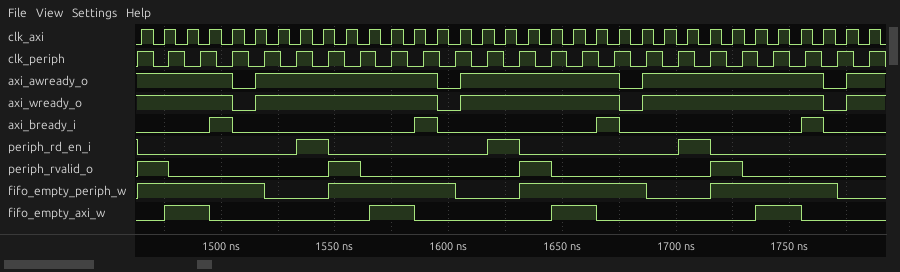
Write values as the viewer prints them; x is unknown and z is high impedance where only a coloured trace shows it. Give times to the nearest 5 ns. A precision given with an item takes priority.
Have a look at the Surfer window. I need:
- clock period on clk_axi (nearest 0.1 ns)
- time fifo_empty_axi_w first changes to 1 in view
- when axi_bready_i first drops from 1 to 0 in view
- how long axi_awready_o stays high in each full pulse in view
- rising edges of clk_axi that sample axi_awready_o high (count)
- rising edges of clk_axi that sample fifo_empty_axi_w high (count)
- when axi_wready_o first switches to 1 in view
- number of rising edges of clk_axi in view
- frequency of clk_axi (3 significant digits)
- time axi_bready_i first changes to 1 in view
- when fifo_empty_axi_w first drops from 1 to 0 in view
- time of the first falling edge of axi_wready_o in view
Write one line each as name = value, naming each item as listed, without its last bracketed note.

clock period on clk_axi = 10 ns
time fifo_empty_axi_w first changes to 1 in view = 1475 ns
when axi_bready_i first drops from 1 to 0 in view = 1505 ns
how long axi_awready_o stays high in each full pulse in view = 80 ns, 70 ns, 80 ns
rising edges of clk_axi that sample axi_awready_o high = 29
rising edges of clk_axi that sample fifo_empty_axi_w high = 8
when axi_wready_o first switches to 1 in view = 1515 ns
number of rising edges of clk_axi in view = 33
frequency of clk_axi = 100 MHz
time axi_bready_i first changes to 1 in view = 1495 ns
when fifo_empty_axi_w first drops from 1 to 0 in view = 1495 ns
time of the first falling edge of axi_wready_o in view = 1505 ns
